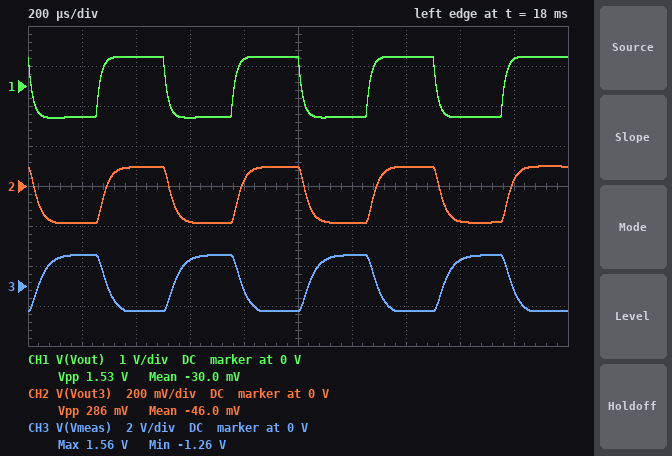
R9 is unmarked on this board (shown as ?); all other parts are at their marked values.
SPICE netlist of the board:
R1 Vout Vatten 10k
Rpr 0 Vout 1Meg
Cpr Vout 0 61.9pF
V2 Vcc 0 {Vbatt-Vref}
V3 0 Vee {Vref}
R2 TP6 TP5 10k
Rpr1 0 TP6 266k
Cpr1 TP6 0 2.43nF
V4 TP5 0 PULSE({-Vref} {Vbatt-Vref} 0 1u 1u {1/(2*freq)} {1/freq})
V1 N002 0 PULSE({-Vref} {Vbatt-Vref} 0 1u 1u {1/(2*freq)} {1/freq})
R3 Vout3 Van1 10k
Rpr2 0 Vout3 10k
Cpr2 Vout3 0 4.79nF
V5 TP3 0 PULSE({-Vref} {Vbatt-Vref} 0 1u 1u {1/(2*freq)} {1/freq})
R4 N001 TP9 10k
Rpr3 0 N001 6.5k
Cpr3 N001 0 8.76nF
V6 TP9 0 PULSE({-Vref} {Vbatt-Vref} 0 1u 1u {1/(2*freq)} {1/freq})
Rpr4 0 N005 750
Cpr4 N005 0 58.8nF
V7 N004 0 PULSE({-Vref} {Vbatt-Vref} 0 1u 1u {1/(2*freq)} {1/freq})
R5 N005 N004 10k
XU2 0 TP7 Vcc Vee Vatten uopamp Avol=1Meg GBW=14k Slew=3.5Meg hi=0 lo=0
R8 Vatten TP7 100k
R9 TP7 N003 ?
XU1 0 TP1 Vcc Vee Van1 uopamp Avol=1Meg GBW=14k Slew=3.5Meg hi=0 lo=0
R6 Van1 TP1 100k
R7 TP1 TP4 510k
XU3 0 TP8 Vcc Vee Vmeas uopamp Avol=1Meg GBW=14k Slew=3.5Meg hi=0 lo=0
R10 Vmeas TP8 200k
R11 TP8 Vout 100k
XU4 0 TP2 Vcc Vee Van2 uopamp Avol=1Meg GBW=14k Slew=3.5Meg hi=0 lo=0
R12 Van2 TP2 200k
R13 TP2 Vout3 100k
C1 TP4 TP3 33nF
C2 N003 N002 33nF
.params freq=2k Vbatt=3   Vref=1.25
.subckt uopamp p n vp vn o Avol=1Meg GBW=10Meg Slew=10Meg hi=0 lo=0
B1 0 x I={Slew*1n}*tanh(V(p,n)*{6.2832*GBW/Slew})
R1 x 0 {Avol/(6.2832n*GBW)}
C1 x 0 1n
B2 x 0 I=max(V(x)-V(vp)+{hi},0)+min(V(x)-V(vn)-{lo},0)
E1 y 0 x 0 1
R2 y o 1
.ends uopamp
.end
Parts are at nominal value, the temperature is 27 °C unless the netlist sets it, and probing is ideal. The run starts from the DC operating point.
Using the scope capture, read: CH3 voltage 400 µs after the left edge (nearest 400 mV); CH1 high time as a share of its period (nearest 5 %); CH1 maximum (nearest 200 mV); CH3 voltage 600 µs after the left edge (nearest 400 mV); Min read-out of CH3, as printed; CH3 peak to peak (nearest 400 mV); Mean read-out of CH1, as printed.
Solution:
-1.2 V
50 %
800 mV
1.2 V
-1.26 V
2.8 V
-30.0 mV
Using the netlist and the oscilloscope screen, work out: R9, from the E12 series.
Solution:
180 kΩ
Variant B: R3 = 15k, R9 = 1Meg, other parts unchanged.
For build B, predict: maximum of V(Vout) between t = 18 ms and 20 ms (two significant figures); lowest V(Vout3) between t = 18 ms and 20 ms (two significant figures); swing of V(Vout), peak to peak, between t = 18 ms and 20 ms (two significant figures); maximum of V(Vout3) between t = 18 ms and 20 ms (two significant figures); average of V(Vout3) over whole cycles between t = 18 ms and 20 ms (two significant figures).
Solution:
64 mV
-150 mV
280 mV
77 mV
-36 mV
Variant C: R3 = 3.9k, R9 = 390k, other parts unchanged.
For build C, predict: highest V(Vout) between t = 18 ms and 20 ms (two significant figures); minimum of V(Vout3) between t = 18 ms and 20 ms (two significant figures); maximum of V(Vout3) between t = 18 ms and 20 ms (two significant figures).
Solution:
280 mV
-280 mV
140 mV
